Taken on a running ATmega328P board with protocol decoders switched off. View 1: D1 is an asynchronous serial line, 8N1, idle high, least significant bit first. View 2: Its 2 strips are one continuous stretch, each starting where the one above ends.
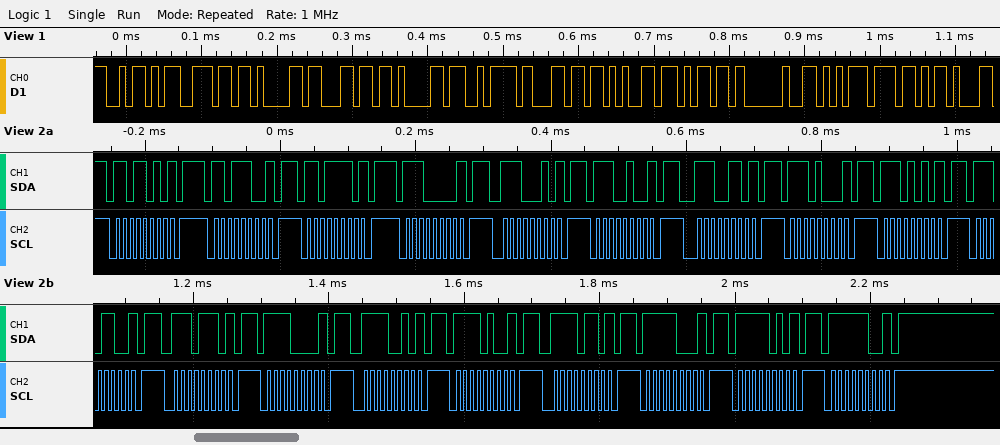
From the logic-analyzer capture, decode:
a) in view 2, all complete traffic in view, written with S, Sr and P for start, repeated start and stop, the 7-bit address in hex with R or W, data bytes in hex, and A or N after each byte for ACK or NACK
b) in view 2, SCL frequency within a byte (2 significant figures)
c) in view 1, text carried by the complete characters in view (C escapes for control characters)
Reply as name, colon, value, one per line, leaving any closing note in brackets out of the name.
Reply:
in view 2, all complete traffic in view, written with S, Sr and P for start, repeated start and stop, the 7-bit address in hex with R or W, data bytes in hex, and A or N after each byte for ACK or NACK: S 6DW N P S 6EW N P S 6FW N P S 70W N P S 71W N P S 72W N P S 73W N P S 74W N P S 75W N P S 76W N P S 77W N P S 78W N P S 79W N P S 7AW N P S 7BW N P S 7CW N P S 7DW N P S 7EW N P
in view 2, SCL frequency within a byte: 100 kHz
in view 1, text carried by the complete characters in view: "Znalazlem uk"
